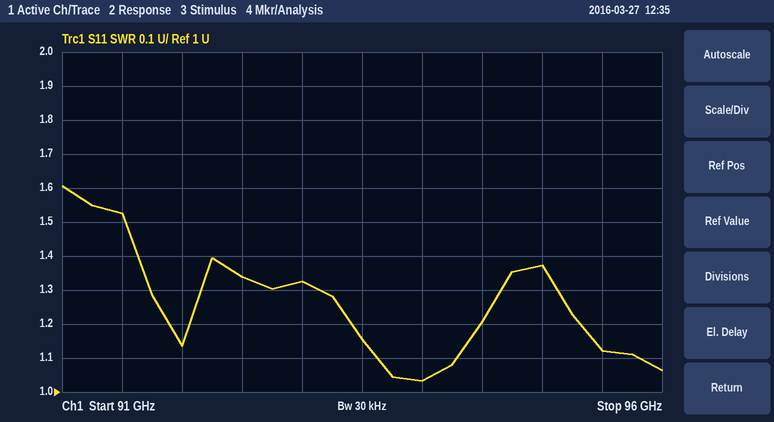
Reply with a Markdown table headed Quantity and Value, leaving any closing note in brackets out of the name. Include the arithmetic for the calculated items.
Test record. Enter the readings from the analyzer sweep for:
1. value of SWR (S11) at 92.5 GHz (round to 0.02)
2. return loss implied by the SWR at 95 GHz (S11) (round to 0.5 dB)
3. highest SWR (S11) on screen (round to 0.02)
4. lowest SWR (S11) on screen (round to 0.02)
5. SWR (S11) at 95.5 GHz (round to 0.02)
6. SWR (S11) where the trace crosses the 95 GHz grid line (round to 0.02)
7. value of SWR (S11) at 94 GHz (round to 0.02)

| Quantity | Value |
|---|---|
| value of SWR (S11) at 92.5 GHz | 1.34 |
| return loss implied by the SWR at 95 GHz (S11) | −20 log10((1.38 − 1)/(1.38 + 1)) ≈ 15.9 dB, so 16.0 dB to the nearest 0.5 dB |
| highest SWR (S11) on screen | 1.60 |
| lowest SWR (S11) on screen | 1.04 |
| SWR (S11) at 95.5 GHz | 1.12 |
| SWR (S11) where the trace crosses the 95 GHz grid line | 1.38 |
| value of SWR (S11) at 94 GHz | 1.04 |
